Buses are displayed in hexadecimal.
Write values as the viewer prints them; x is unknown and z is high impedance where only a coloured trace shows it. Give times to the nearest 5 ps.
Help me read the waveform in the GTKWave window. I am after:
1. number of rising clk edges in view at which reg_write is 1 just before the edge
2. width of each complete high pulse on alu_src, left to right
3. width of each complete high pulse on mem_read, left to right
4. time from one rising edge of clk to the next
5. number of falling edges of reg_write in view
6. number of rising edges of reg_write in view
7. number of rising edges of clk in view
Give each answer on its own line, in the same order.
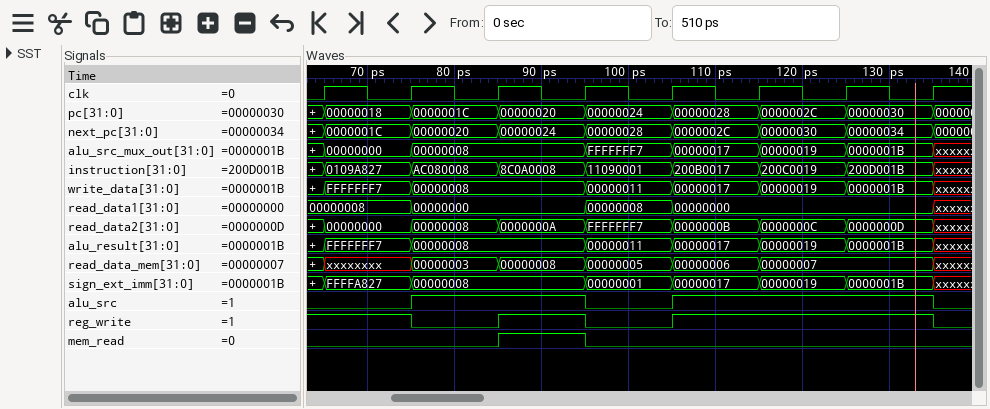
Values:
6
20 ps, 30 ps
10 ps
10 ps
3
2
8
